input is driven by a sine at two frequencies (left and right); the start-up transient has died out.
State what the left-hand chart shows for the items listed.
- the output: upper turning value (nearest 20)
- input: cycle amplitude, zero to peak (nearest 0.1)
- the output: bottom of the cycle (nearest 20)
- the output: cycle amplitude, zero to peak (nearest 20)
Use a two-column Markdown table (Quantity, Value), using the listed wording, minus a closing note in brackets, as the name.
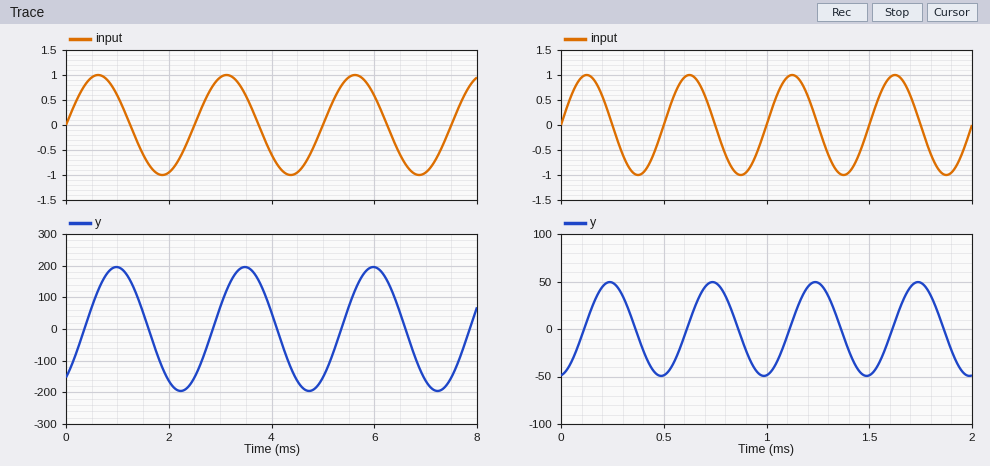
| Quantity | Value |
|---|---|
| the output: upper turning value | 200 |
| input: cycle amplitude, zero to peak | 1.0 |
| the output: bottom of the cycle | -200 |
| the output: cycle amplitude, zero to peak | 200 |
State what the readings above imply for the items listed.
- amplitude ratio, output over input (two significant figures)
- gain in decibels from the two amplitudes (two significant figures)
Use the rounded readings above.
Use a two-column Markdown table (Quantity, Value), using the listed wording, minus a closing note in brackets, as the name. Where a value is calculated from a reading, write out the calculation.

| Quantity | Value |
|---|---|
| amplitude ratio, output over input | 200 / 1 = 200 |
| gain in decibels from the two amplitudes | 20 log10(200 / 1) = 46 dB |
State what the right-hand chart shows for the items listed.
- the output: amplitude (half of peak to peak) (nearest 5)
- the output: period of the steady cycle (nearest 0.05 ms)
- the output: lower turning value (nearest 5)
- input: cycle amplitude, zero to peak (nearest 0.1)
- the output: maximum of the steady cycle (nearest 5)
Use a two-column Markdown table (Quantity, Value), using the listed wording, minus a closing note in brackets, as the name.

| Quantity | Value |
|---|---|
| the output: amplitude (half of peak to peak) | 50 |
| the output: period of the steady cycle | 0.50 ms |
| the output: lower turning value | -50 |
| input: cycle amplitude, zero to peak | 1.0 |
| the output: maximum of the steady cycle | 50 |
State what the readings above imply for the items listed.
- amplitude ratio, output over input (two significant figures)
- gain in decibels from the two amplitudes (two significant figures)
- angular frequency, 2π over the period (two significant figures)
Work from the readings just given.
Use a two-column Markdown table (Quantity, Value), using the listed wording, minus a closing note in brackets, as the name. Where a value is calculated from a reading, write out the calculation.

| Quantity | Value |
|---|---|
| amplitude ratio, output over input | 50 / 1 = 50 |
| gain in decibels from the two amplitudes | 20 log10(50 / 1) = 34 dB |
| angular frequency, 2π over the period | 2π / 0.5 = 13 rad/ms |
